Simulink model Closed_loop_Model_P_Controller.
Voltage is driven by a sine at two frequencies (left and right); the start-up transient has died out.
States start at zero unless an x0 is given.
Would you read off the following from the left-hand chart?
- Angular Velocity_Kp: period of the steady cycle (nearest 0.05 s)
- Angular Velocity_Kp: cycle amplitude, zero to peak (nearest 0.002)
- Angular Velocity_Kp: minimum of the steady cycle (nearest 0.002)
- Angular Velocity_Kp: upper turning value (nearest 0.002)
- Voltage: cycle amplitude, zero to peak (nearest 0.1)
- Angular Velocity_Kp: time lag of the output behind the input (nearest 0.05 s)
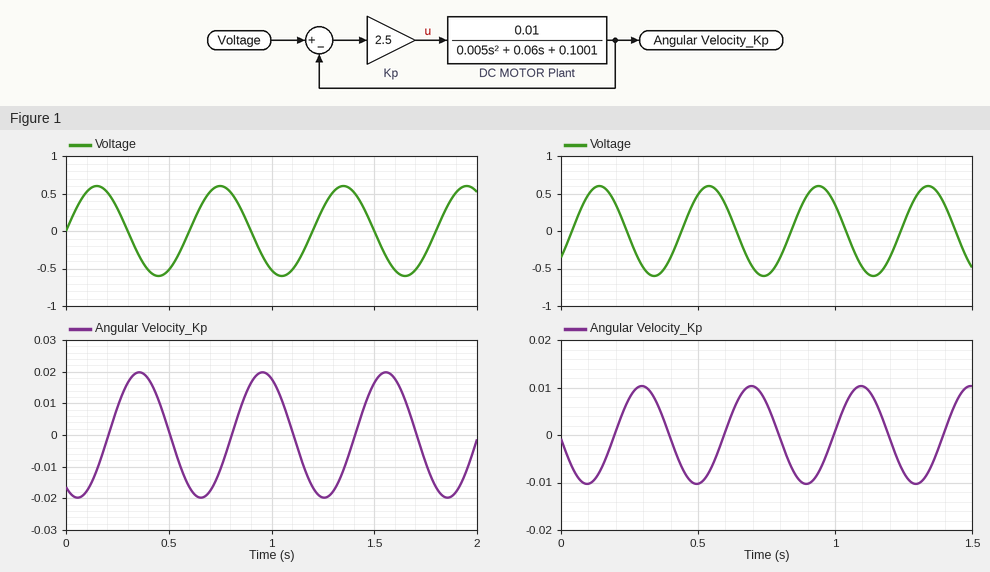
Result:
0.60 s
0.020
-0.020
0.020
0.6
0.20 s
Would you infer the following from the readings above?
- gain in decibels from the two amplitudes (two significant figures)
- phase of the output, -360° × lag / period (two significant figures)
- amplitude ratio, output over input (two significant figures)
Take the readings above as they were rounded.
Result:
-30 dB
-120°
0.033
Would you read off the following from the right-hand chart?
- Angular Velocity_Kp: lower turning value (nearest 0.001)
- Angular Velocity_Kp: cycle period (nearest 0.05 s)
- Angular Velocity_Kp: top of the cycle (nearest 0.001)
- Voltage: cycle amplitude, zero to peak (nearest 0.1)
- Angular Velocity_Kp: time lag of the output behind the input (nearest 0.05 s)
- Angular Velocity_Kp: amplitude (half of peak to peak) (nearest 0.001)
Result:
-0.010
0.40 s
0.010
0.6
0.15 s
0.010
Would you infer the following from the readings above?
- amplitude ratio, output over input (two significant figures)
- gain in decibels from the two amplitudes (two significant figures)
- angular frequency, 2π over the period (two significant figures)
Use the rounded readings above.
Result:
0.017
-36 dB
16 rad/s
